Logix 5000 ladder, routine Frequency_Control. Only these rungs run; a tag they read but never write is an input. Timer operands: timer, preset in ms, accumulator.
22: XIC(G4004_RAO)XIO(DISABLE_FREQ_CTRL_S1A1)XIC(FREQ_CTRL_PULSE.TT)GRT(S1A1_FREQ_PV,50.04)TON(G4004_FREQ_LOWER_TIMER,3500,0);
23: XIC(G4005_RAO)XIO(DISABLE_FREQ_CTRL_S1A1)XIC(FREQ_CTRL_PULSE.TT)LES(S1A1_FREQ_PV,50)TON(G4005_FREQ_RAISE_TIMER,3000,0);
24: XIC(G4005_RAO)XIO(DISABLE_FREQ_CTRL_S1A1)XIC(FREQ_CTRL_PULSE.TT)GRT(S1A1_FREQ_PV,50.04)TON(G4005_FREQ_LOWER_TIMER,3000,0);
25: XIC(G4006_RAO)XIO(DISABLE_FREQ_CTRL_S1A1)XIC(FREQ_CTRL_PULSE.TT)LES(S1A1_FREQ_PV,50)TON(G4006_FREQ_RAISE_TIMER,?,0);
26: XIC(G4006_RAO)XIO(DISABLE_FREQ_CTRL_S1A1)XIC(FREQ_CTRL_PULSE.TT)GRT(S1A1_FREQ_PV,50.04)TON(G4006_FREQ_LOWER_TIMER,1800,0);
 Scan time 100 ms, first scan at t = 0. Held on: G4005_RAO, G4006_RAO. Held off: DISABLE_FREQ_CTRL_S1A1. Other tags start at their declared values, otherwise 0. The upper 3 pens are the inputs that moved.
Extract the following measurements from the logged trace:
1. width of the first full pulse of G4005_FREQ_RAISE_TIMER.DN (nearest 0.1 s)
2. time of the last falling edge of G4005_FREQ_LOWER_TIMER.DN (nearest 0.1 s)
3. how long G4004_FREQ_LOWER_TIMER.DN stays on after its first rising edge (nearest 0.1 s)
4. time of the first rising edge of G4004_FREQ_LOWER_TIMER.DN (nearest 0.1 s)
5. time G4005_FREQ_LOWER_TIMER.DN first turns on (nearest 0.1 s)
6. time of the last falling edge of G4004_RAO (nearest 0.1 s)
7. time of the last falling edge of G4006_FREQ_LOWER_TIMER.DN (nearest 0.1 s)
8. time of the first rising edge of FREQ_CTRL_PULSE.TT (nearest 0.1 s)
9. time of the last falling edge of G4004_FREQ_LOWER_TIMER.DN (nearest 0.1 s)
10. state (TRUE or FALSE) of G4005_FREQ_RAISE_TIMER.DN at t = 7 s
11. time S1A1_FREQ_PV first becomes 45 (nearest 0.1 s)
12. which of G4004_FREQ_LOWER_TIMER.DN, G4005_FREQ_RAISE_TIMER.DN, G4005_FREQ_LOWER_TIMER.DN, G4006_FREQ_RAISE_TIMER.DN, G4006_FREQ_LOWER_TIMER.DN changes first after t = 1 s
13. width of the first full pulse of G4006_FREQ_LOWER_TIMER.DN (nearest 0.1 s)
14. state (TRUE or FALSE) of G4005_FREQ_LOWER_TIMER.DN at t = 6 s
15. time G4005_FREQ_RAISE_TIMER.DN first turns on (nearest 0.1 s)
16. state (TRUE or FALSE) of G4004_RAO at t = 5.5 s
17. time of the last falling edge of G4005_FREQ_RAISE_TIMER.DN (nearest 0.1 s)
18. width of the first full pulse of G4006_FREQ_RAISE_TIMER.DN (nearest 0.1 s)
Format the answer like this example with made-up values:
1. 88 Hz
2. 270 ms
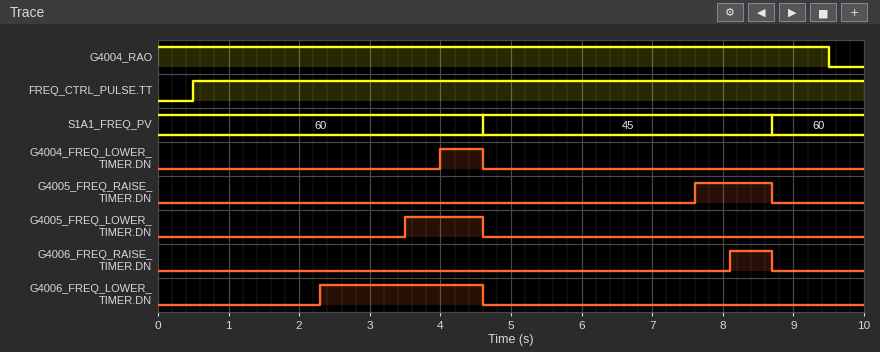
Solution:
1. 1.1 s
2. 4.6 s
3. 0.6 s
4. 4.0 s
5. 3.5 s
6. 9.5 s
7. 4.6 s
8. 0.5 s
9. 4.6 s
10. FALSE
11. 4.6 s
12. G4006_FREQ_LOWER_TIMER.DN
13. 2.3 s
14. FALSE
15. 7.6 s
16. TRUE
17. 8.7 s
18. 0.6 s
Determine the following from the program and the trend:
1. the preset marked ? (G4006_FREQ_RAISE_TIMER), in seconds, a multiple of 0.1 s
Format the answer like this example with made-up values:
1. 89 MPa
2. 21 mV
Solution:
1. 3.5 s
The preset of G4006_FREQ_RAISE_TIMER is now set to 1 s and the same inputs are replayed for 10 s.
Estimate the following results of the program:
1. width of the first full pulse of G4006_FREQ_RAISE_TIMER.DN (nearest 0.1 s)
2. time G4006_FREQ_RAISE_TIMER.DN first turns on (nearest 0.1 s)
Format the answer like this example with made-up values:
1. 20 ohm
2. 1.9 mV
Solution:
1. 3.1 s
2. 5.6 s
